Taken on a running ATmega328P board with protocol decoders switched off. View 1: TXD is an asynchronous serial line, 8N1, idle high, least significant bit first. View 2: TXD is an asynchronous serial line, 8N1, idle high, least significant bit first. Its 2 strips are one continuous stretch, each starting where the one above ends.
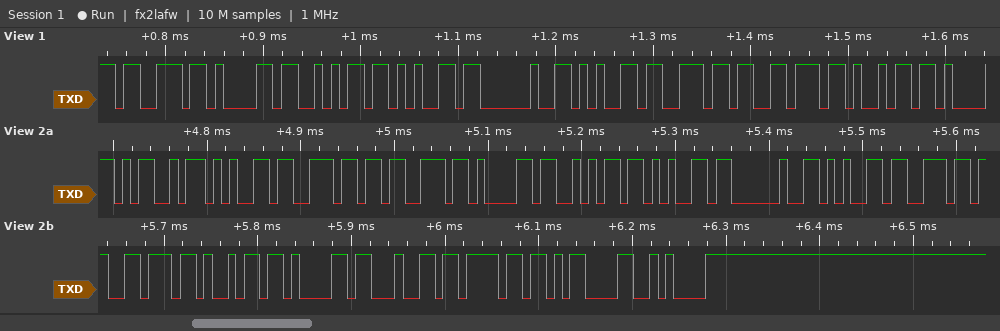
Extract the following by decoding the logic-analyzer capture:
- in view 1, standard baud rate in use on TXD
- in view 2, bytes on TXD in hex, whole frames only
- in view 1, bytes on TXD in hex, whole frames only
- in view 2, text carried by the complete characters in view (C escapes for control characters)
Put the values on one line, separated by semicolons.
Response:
115200 baud; 0x4D 0x65 0x6E 0x73 0x61 0x6A 0x65 0x20 0x65 0x6E 0x76 0x69 0x61 0x64 0x6F 0x0D 0x0A; 0x73 0x61 0x6A 0x65 0x20 0x65 0x6E 0x76 0x69; "Mensaje enviado\r\n"
